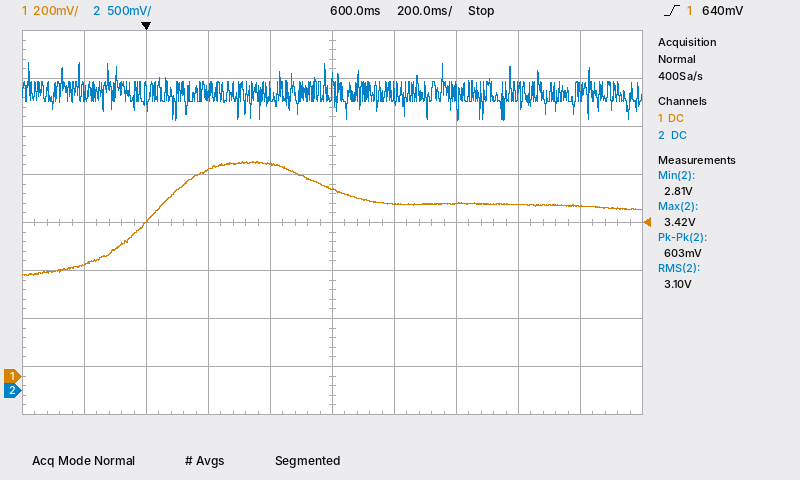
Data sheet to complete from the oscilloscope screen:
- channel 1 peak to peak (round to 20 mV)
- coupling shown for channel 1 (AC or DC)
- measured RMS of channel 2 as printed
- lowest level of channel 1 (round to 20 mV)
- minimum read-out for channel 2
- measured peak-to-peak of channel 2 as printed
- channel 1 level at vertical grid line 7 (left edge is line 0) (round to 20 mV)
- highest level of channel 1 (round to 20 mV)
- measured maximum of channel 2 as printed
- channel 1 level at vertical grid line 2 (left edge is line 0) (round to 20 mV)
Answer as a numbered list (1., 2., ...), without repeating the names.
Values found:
1. 480 mV
2. DC
3. 3.10 V
4. 420 mV
5. 2.81 V
6. 603 mV
7. 720 mV
8. 900 mV
9. 3.42 V
10. 640 mV
